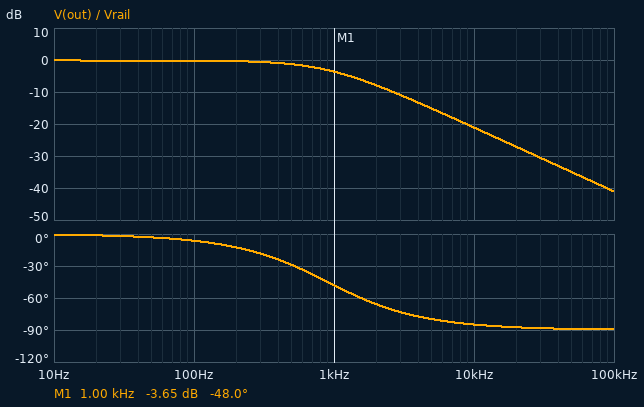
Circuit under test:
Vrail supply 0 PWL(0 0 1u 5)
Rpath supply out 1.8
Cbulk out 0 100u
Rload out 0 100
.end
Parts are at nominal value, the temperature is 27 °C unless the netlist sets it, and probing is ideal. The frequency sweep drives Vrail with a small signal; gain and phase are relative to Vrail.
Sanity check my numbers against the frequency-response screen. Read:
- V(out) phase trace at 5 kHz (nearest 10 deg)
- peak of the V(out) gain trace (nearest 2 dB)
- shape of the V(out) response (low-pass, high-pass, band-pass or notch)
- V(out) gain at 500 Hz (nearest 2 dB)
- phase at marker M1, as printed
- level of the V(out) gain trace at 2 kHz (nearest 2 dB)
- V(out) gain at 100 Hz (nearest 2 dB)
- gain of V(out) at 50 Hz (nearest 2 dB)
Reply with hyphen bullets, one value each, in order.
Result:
- -80 deg
- 0 dB
- low-pass
- -2 dB
- -48.0 deg
- -8 dB
- 0 dB
- 0 dB
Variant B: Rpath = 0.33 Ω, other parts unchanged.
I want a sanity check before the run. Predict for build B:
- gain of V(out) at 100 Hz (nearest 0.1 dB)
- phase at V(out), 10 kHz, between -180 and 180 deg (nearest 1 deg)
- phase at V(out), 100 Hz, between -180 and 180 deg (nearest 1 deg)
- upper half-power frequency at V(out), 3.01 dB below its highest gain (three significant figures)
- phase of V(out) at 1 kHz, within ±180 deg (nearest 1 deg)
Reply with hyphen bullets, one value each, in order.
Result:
- 0 dB
- -64 deg
- -1 deg
- 4.84 kHz
- -12 deg
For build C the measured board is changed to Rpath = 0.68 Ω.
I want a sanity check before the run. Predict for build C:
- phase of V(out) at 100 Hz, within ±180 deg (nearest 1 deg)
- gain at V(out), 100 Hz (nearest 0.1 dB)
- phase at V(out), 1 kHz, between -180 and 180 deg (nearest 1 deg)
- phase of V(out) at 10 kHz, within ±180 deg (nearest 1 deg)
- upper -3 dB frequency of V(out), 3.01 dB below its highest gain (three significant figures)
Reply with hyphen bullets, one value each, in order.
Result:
- -2 deg
- -0.1 dB
- -23 deg
- -77 deg
- 2.36 kHz
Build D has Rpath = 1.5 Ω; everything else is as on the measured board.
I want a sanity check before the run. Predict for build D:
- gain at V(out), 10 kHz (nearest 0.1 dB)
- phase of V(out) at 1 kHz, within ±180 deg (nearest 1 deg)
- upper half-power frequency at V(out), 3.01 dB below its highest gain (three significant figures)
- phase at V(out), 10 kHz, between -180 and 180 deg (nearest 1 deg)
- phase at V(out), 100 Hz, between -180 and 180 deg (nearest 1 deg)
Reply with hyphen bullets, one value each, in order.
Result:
- -19.5 dB
- -43 deg
- 1.08 kHz
- -84 deg
- -5 deg
